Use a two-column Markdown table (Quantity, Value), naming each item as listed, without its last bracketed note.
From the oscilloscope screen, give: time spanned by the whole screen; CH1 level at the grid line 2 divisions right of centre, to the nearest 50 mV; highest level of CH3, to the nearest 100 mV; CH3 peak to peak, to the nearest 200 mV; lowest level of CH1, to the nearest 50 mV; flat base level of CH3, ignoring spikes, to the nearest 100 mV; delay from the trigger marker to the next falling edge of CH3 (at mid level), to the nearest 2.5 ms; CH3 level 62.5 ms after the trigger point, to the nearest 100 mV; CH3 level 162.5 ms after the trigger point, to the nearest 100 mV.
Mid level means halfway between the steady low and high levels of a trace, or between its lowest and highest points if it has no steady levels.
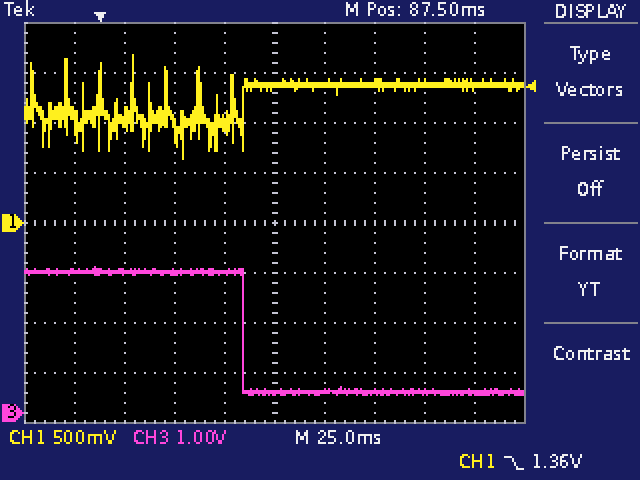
| Quantity | Value |
|---|---|
| time spanned by the whole screen | 250 ms |
| CH1 level at the grid line 2 divisions right of centre, to the nearest 50 mV | 1.40 V |
| highest level of CH3, to the nearest 100 mV | 2.9 V |
| CH3 peak to peak, to the nearest 200 mV | 2.6 V |
| lowest level of CH1, to the nearest 50 mV | 650 mV |
| flat base level of CH3, ignoring spikes, to the nearest 100 mV | 400 mV |
| delay from the trigger marker to the next falling edge of CH3 (at mid level), to the nearest 2.5 ms | 72.5 ms |
| CH3 level 62.5 ms after the trigger point, to the nearest 100 mV | 2.8 V |
| CH3 level 162.5 ms after the trigger point, to the nearest 100 mV | 400 mV |
